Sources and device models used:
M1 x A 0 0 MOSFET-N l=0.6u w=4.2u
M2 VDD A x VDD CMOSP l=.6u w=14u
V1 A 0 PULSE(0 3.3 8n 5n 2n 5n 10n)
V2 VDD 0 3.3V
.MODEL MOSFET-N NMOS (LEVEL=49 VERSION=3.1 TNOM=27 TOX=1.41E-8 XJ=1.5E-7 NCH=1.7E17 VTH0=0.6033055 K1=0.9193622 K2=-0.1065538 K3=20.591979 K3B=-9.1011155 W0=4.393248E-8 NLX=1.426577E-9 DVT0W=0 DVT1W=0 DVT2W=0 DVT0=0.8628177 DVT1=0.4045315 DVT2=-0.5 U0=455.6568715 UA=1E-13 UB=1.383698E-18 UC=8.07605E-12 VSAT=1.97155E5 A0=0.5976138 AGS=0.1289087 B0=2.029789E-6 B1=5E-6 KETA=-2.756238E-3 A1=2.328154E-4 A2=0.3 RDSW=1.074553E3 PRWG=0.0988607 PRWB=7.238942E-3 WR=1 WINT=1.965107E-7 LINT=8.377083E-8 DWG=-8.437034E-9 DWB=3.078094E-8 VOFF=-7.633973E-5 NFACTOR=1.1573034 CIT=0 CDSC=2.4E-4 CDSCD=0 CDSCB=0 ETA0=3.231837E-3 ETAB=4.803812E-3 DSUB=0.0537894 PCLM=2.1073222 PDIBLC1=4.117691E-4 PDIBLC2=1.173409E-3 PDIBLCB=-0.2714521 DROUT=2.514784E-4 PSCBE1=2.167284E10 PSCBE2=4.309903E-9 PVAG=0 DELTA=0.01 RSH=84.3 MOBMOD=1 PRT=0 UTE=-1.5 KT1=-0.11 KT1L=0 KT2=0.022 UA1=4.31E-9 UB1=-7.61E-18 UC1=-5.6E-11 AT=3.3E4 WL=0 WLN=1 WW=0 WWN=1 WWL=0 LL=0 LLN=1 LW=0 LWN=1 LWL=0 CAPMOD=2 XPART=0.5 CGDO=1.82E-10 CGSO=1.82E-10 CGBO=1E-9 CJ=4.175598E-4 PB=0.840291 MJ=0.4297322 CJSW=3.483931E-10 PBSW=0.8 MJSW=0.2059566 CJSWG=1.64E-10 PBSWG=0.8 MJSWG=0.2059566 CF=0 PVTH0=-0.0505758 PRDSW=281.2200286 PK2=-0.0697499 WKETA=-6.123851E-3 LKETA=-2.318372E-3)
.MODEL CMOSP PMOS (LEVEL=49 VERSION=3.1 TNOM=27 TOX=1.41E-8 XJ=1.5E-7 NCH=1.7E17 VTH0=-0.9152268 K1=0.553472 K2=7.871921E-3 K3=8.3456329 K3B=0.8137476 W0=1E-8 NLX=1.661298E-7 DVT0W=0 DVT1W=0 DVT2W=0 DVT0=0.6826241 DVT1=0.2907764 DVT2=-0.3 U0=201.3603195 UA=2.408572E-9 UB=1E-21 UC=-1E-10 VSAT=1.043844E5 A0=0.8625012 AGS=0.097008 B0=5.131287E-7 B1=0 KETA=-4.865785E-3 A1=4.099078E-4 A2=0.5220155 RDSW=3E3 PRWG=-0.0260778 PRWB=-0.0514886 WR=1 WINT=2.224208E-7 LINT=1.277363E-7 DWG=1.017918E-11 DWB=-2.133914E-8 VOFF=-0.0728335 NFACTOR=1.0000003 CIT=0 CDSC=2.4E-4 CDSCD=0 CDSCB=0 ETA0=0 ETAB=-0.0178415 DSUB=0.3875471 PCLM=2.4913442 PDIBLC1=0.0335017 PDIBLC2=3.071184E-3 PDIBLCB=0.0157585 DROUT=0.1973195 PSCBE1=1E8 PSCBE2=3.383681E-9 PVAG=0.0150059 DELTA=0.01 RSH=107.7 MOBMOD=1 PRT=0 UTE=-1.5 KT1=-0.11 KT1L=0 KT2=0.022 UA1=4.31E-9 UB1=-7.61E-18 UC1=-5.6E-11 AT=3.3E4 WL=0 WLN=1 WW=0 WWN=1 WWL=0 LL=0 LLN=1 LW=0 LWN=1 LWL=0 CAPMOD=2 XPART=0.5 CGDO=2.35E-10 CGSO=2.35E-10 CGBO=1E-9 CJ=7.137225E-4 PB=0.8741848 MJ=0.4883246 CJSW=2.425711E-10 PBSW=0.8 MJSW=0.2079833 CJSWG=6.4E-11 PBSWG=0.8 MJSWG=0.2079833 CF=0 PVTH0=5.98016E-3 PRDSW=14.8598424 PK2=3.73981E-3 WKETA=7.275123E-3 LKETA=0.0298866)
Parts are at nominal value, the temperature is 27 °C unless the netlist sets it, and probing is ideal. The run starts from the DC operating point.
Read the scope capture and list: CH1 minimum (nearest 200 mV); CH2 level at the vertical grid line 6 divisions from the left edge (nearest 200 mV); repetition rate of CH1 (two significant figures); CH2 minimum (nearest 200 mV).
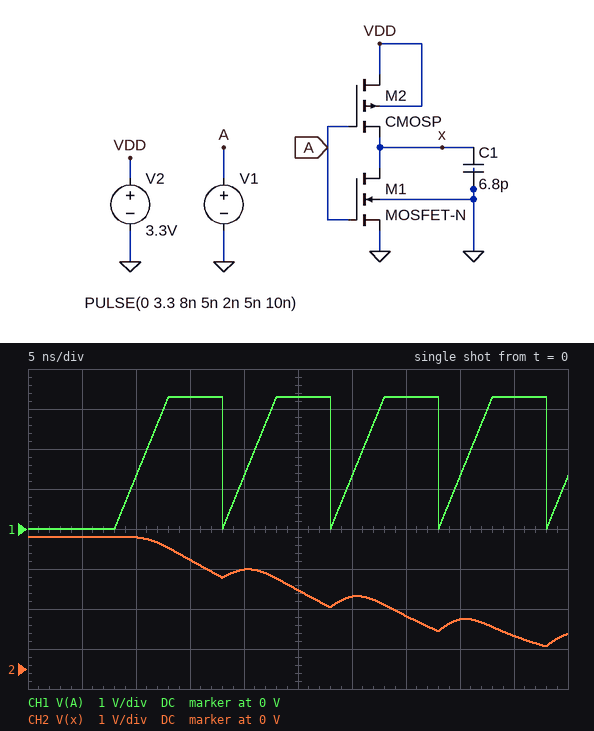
0 V
1.8 V
100 MHz
600 mV
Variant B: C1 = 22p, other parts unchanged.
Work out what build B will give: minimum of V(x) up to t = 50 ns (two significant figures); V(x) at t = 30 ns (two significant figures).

2.2 V
2.7 V
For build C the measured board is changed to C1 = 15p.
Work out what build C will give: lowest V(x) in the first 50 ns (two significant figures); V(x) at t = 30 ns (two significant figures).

1.8 V
2.5 V
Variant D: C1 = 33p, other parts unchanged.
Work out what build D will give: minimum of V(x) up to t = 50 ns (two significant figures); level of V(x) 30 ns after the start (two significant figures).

2.5 V
2.9 V
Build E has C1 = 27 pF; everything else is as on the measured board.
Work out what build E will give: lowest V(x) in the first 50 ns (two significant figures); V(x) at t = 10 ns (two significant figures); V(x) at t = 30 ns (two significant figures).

2.4 V
3.3 V
2.8 V
